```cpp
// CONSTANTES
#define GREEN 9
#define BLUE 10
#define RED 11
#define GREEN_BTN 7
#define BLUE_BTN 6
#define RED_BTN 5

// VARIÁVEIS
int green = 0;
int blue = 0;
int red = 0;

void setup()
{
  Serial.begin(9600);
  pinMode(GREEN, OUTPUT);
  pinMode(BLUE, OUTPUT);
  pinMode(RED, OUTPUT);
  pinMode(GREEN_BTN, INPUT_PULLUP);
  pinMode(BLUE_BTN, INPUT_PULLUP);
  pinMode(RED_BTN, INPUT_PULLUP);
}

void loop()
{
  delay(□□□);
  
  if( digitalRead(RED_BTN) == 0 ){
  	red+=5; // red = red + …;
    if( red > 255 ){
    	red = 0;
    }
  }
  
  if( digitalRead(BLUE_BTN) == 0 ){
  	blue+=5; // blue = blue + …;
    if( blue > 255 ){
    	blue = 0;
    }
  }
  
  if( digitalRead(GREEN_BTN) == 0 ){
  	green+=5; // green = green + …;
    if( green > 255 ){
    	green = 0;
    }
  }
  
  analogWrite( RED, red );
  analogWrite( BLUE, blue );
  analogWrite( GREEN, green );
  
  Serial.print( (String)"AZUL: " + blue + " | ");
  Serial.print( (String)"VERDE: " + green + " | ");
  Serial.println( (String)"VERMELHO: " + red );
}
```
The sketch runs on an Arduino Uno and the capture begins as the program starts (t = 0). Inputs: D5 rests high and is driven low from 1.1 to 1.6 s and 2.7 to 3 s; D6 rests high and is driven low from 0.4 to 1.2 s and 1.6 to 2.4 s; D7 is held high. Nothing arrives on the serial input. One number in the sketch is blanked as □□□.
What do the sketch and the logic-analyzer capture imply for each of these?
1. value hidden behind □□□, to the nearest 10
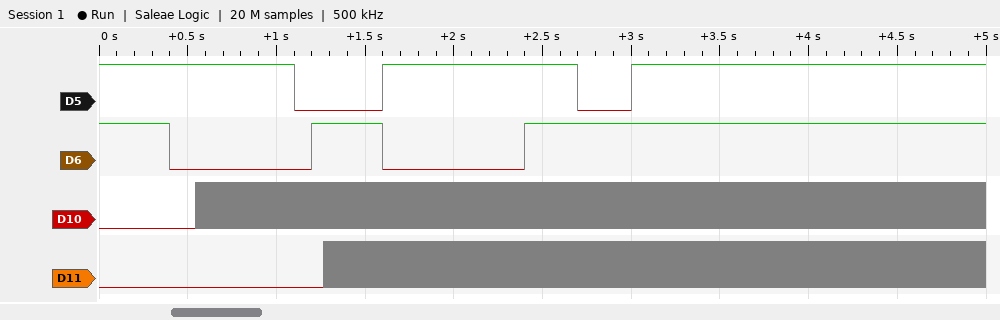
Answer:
180
